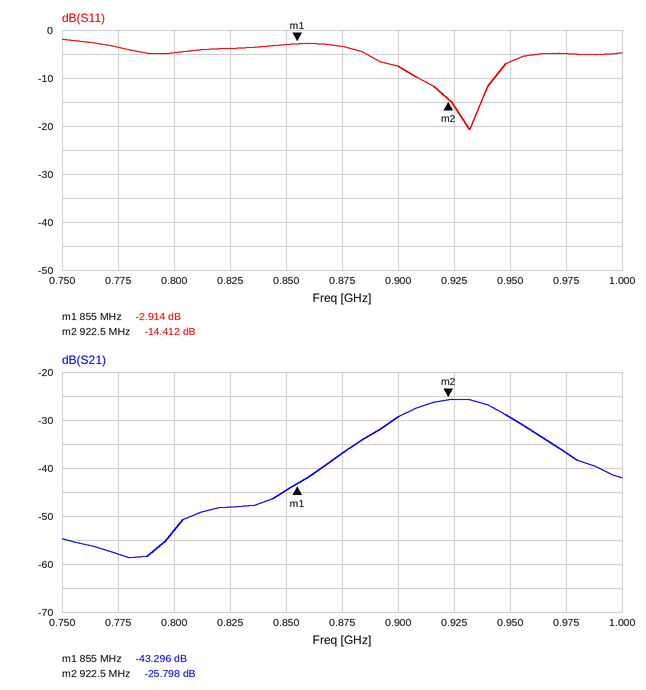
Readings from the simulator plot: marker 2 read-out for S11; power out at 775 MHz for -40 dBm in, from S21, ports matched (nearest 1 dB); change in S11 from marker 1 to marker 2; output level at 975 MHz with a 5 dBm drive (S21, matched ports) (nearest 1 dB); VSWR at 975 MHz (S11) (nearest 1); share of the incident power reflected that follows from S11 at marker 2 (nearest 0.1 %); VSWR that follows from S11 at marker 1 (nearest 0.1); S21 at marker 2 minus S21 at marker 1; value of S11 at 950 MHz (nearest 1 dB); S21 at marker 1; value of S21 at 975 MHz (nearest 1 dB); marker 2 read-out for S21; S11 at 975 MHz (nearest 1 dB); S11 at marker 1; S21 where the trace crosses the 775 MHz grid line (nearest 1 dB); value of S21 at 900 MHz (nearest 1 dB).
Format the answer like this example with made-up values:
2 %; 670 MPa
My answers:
-14.412 dB; -98 dBm; -11.498 dB; -32 dBm; 4; 3.6 %; 6.0; 17.498 dB; -7 dB; -43.296 dB; -37 dB; -25.798 dB; -5 dB; -2.914 dB; -58 dB; -29 dB
